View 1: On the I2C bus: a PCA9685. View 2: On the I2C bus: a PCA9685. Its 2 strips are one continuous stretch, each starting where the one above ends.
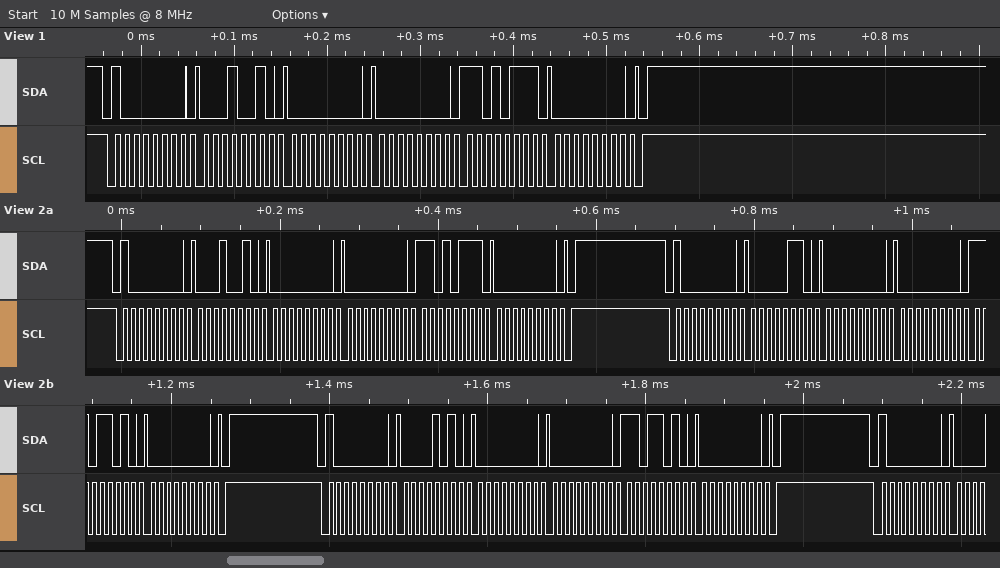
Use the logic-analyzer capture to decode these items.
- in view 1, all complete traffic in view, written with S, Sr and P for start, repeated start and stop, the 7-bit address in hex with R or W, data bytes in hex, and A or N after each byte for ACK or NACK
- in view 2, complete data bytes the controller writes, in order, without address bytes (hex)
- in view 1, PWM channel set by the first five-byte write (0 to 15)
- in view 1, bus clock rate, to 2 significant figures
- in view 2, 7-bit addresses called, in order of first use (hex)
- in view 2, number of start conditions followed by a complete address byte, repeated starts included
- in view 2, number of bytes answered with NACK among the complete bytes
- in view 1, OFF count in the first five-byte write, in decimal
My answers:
S 40W A 12 A 00 A 00 A D7 A 00 A P
12 00 00 D7 00 06 00 00 DA 00 0A 00 00 DA 00
3
100 kHz
0x40
4
0
215
